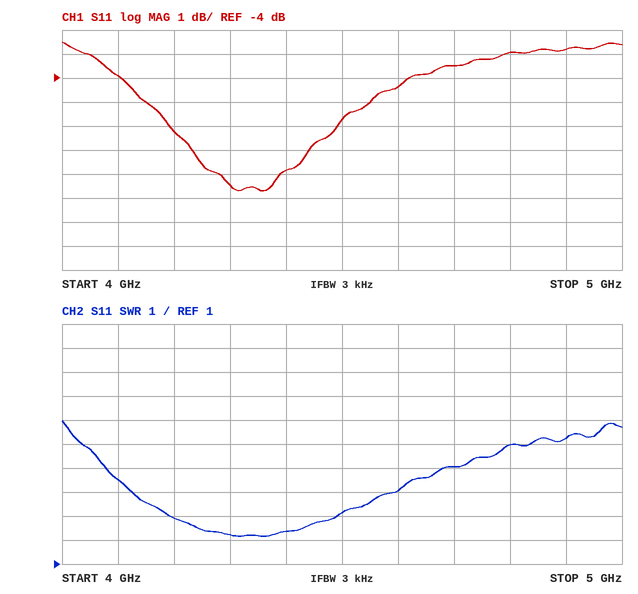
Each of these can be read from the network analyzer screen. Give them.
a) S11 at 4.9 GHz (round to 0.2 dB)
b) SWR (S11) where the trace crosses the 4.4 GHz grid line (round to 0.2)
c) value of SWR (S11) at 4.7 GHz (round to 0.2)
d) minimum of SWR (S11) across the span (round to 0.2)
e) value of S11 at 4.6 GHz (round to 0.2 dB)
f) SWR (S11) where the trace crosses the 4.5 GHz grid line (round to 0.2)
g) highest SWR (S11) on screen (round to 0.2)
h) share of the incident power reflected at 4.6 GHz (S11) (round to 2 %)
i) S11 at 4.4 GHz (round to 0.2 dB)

-2.8 dB
2.4
5.0
2.2
-4.4 dB
3.2
7.0
36 %
-7.8 dB
